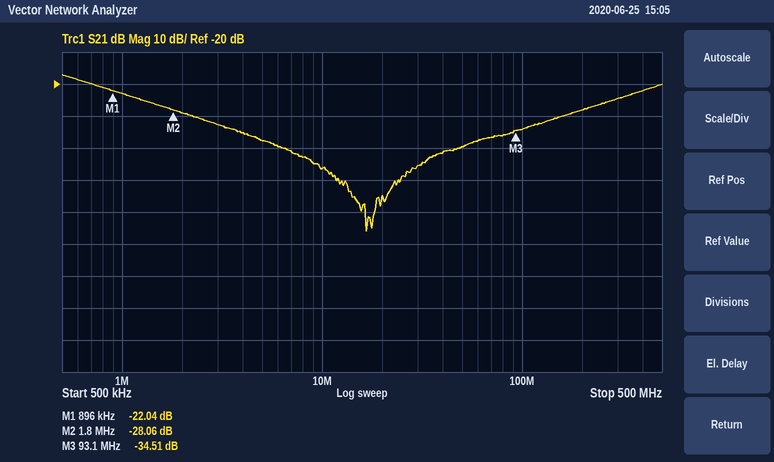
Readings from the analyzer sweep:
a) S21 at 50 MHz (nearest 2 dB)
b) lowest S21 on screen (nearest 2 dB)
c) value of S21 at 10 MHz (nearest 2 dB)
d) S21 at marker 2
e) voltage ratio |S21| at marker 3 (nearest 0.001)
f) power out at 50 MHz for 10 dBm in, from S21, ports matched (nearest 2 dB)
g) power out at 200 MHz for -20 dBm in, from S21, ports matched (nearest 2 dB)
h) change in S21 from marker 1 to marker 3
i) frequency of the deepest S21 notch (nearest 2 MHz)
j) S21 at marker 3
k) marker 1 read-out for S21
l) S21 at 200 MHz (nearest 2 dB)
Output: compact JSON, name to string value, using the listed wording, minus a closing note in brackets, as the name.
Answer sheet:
{"S21 at 50 MHz": "-40 dB", "lowest S21 on screen": "-66 dB", "value of S21 at 10 MHz": "-46 dB", "S21 at marker 2": "-28.06 dB", "voltage ratio |S21| at marker 3": "0.019", "power out at 50 MHz for 10 dBm in, from S21, ports matched": "-30 dBm", "power out at 200 MHz for -20 dBm in, from S21, ports matched": "-48 dBm", "change in S21 from marker 1 to marker 3": "-12.47 dB", "frequency of the deepest S21 notch": "16 MHz", "S21 at marker 3": "-34.51 dB", "marker 1 read-out for S21": "-22.04 dB", "S21 at 200 MHz": "-28 dB"}
